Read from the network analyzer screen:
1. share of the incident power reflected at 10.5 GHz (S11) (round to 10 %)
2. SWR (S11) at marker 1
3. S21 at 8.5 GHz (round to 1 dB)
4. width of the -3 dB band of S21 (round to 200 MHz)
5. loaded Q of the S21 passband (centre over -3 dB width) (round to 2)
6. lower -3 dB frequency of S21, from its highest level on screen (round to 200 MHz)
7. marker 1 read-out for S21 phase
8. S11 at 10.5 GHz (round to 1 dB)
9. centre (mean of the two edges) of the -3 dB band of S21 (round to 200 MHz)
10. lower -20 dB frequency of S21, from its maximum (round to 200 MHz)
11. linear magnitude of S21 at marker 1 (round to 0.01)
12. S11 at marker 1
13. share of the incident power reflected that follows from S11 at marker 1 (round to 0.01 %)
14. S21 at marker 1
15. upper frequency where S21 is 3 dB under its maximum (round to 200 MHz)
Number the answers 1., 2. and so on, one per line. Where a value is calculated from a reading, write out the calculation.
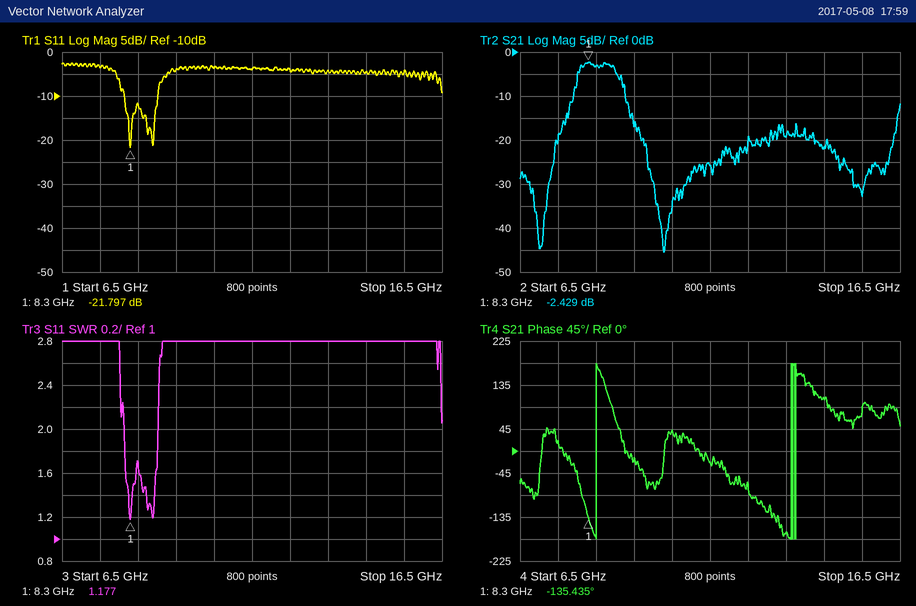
1. 10^(-4/10) ≈ 40 %
2. 1.177
3. -3 dB
4. 9.0 GHz − 8.0 GHz = 1.0 GHz
5. 8.5 GHz / 1 GHz ≈ 8
6. 8.0 GHz
7. -135.435°
8. -4 dB
9. 8.6 GHz
10. 7.4 GHz
11. 10^(-2.429/20) ≈ 0.76
12. -21.797 dB
13. 10^(-21.797/10) ≈ 0.66 %
14. -2.429 dB
15. 9.0 GHz
